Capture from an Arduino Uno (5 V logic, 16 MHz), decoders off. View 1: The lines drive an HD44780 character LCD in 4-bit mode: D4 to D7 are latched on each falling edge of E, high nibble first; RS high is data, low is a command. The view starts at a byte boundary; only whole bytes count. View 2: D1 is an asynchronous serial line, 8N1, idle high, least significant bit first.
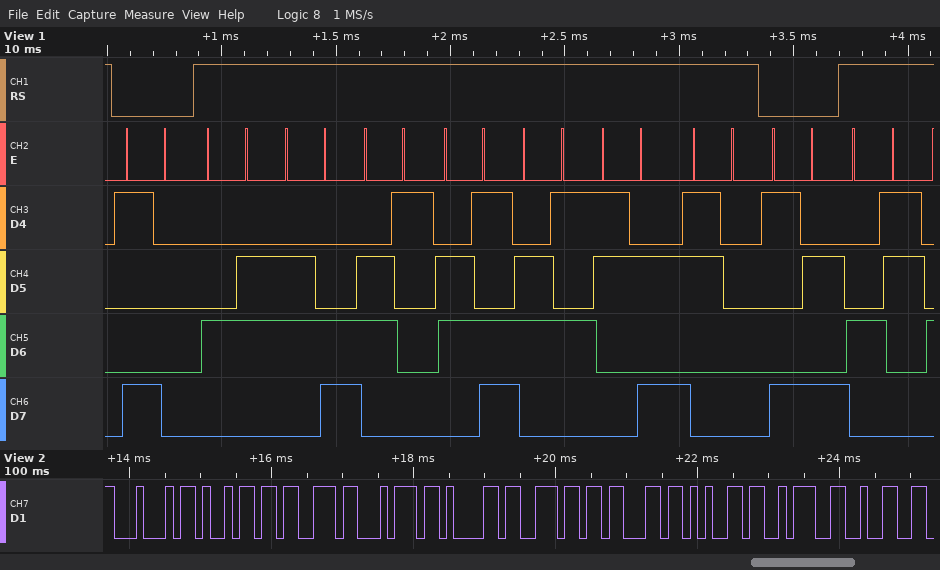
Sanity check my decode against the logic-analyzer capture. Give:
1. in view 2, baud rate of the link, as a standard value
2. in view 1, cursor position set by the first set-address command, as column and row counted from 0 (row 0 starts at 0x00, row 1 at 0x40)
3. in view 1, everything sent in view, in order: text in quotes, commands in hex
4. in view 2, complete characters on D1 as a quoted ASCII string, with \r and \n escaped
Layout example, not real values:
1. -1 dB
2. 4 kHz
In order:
1. 9600 baud
2. column 16, row 0
3. 0x90 "Flame:0" 0x9A "C"
4. "Distance:2"
